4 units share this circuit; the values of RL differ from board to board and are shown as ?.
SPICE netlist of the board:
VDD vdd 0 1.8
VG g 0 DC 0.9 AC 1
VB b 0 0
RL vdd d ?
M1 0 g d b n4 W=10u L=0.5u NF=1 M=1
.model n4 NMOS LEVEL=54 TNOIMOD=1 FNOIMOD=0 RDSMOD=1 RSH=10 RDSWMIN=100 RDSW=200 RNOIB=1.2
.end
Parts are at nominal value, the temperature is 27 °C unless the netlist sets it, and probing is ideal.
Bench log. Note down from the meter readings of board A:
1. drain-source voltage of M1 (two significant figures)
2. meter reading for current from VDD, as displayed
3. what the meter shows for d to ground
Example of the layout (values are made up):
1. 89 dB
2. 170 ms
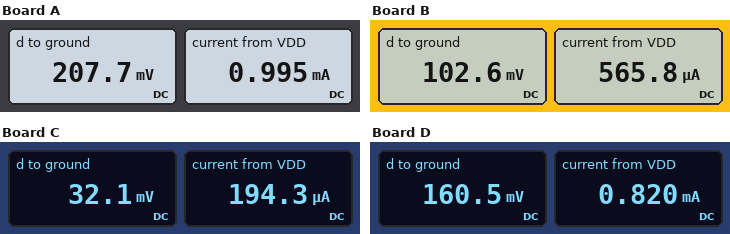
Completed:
1. -210 mV
2. 0.995 mA
3. 207.7 mV
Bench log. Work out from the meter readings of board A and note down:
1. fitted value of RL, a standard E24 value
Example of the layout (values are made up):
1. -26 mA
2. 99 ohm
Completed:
1. 1.6 kΩ
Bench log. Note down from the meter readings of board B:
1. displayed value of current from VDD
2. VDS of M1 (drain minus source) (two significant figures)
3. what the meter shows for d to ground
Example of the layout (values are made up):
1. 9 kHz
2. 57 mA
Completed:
1. 565.8 µA
2. -100 mV
3. 102.6 mV
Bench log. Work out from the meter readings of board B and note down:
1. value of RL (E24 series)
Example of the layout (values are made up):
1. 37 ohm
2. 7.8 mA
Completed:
1. 3 kΩ
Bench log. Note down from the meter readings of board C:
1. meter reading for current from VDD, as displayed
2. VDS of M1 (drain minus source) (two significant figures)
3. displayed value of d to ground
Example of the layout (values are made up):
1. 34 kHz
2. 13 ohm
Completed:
1. 194.3 µA
2. -32 mV
3. 32.1 mV
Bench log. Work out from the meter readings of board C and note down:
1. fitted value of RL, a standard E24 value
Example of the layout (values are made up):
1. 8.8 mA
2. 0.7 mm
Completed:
1. 9.1 kΩ
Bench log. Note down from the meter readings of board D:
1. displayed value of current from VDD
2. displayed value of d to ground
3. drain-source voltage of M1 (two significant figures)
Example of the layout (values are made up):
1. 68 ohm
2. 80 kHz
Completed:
1. 0.820 mA
2. 160.5 mV
3. -160 mV
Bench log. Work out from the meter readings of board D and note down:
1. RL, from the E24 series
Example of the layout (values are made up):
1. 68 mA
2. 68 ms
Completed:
1. 2 kΩ
